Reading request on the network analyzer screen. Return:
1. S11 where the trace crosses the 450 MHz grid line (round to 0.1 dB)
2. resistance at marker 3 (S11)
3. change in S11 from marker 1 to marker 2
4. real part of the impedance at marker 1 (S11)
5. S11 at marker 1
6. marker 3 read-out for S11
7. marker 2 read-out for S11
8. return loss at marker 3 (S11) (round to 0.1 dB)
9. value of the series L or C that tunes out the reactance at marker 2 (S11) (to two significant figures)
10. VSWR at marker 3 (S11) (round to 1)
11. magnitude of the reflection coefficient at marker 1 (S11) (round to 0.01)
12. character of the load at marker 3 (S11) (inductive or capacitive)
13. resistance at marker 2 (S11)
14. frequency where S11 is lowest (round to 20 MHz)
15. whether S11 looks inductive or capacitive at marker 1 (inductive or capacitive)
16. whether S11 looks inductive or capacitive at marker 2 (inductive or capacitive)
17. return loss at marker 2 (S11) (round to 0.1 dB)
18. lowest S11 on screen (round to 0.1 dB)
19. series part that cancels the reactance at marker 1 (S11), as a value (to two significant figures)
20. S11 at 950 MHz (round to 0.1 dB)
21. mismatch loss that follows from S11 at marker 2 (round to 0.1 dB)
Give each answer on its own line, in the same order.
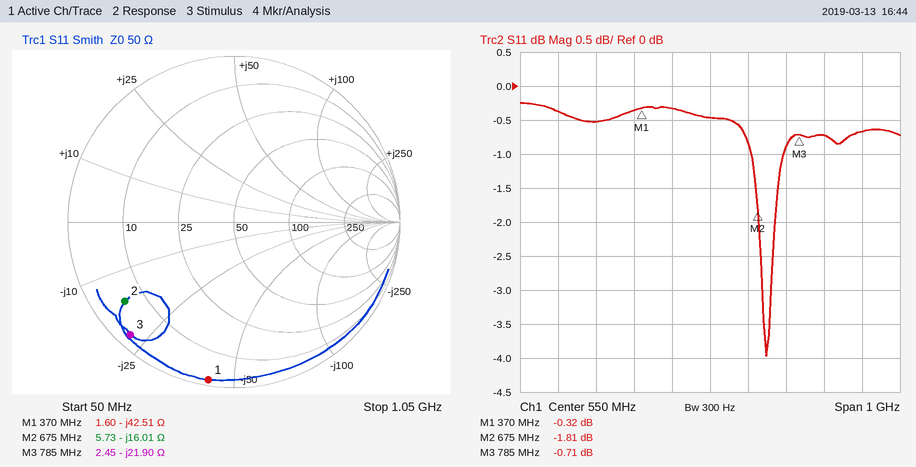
-0.3 dB
2.45 Ω
-1.49 dB
1.60 Ω
-0.32 dB
-0.71 dB
-1.81 dB
0.7 dB
3.8 nH
24
0.96
capacitive
5.73 Ω
700 MHz
capacitive
capacitive
1.8 dB
-4.0 dB
18 nH
-0.7 dB
4.7 dB
